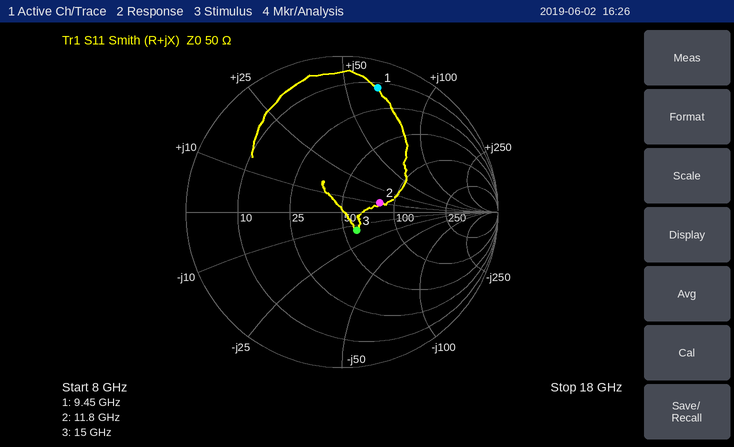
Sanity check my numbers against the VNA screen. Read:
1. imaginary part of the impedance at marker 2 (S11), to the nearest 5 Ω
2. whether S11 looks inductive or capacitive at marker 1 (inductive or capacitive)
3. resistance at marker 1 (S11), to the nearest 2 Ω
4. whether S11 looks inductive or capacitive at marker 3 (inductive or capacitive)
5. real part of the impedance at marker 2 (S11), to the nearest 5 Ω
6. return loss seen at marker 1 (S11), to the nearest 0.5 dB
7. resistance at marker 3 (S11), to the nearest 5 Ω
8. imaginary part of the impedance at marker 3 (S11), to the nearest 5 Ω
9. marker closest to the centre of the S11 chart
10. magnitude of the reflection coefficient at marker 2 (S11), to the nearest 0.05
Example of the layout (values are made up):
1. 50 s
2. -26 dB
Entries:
1. +10 Ω
2. inductive
3. 12 Ω
4. capacitive
5. 80 Ω
6. 1.5 dB
7. 60 Ω
8. -15 Ω
9. marker 3
10. 0.25
